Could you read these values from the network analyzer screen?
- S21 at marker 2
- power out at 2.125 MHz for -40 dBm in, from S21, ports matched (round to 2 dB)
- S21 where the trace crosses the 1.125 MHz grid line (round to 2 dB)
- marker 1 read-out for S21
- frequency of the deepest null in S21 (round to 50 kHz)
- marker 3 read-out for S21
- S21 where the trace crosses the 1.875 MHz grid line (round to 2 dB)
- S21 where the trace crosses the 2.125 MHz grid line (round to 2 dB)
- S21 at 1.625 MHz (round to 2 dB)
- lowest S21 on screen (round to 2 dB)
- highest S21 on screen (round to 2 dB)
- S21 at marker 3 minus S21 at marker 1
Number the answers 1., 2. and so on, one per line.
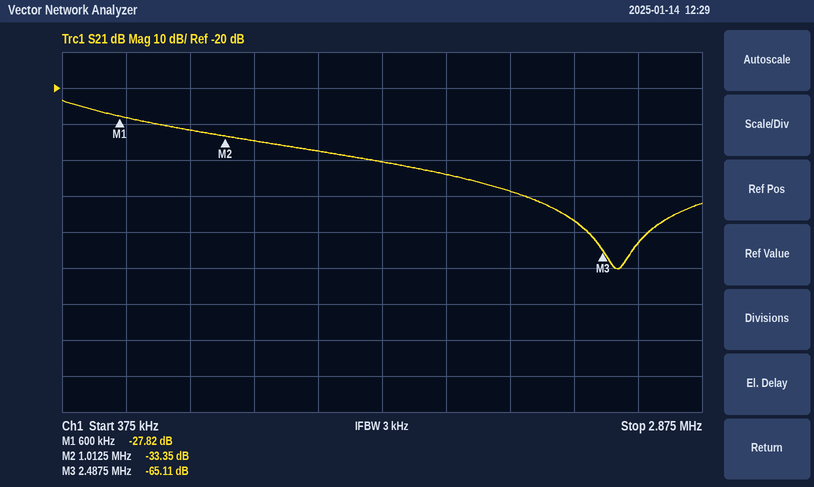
1. -33.35 dB
2. -88 dBm
3. -34 dB
4. -27.82 dB
5. 2.55 MHz
6. -65.11 dB
7. -44 dB
8. -48 dB
9. -40 dB
10. -70 dB
11. -24 dB
12. -37.29 dB
